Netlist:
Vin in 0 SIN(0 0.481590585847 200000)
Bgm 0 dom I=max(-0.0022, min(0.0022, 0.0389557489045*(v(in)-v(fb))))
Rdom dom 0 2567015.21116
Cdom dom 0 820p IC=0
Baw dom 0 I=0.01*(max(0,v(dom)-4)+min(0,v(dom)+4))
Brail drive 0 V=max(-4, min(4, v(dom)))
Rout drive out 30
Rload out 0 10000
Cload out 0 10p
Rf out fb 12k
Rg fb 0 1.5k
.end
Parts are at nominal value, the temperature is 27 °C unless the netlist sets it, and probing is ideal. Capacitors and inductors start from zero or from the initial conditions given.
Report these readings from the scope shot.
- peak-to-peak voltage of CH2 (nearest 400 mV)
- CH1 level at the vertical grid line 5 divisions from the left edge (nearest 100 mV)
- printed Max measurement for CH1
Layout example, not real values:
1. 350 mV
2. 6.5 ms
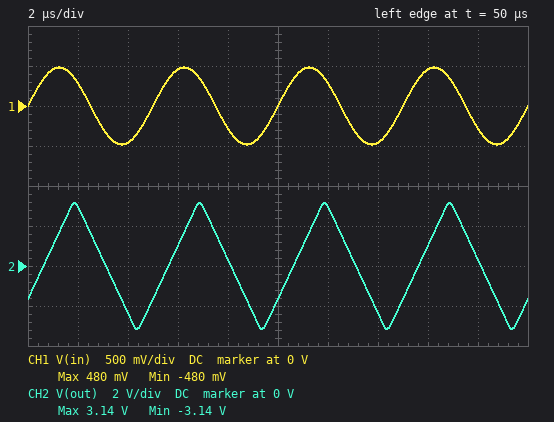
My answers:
1. 6.4 V
2. 0 V
3. 480 mV
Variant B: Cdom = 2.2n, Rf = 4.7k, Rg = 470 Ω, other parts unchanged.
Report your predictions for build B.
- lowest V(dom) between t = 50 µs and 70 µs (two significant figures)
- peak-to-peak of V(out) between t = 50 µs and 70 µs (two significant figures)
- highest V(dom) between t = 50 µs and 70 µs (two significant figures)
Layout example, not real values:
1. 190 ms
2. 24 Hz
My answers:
1. -1.2 V
2. 2.4 V
3. 1.2 V
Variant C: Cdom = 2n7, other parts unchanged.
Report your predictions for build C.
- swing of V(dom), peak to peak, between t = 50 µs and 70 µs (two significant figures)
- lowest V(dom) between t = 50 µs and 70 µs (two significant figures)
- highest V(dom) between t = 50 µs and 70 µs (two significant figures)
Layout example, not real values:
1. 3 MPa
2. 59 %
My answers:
1. 2.0 V
2. -980 mV
3. 980 mV
